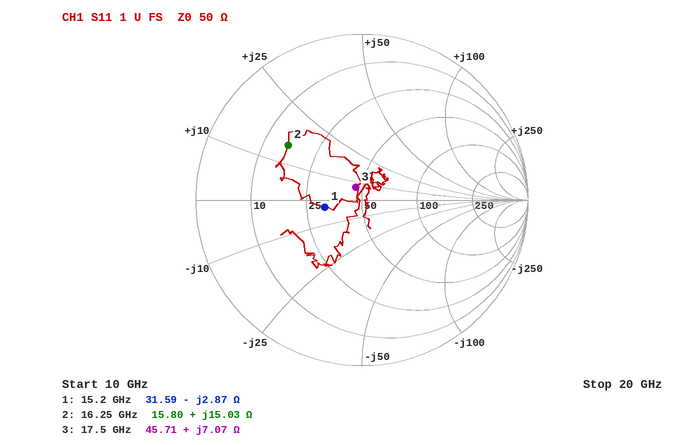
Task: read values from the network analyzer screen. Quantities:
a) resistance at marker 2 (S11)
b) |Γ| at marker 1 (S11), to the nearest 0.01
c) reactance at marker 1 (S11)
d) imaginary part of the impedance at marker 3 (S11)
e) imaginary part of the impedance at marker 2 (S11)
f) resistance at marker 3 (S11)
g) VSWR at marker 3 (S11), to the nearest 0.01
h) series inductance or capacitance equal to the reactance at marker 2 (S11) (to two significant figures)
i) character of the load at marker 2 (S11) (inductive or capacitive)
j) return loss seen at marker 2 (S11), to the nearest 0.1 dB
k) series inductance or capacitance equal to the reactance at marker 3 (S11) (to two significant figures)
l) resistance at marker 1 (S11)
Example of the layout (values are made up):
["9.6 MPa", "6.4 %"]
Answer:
["15.80 Ω", "0.23", "-2.87 Ω", "+7.07 Ω", "+15.03 Ω", "45.71 Ω", "1.19", "150 pH", "inductive", "5.1 dB", "64 pH", "31.59 Ω"]
